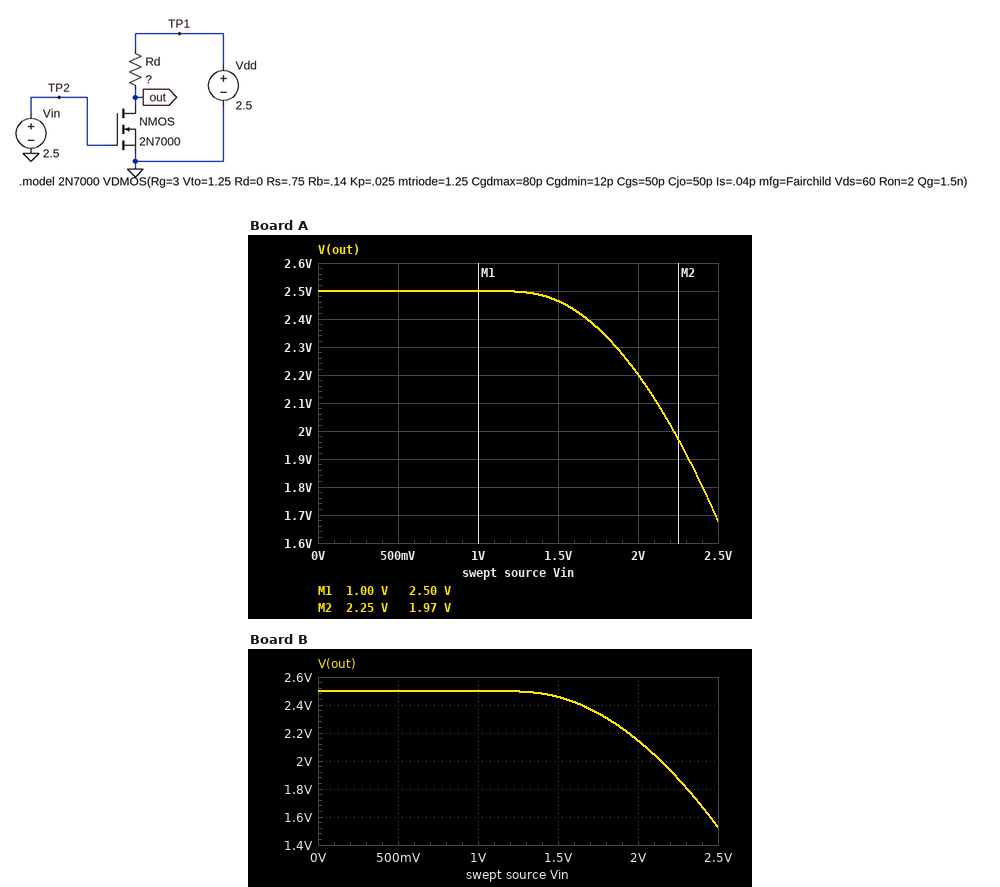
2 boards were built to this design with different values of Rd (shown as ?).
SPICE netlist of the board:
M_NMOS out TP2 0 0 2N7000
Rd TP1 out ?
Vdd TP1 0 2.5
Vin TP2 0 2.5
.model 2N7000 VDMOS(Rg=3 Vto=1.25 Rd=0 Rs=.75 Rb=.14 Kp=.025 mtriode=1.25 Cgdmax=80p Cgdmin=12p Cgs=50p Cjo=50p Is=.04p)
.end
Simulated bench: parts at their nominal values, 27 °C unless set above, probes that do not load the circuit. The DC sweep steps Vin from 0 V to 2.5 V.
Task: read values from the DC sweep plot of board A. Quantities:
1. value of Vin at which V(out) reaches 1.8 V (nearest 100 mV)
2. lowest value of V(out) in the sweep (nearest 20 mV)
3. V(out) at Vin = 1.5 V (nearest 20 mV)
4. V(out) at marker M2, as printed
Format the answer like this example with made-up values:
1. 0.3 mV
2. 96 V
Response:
1. 2.4 V
2. 1.68 V
3. 2.46 V
4. 1.97 V
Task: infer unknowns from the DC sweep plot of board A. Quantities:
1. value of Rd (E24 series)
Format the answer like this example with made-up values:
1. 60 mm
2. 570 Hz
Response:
1. 43 Ω
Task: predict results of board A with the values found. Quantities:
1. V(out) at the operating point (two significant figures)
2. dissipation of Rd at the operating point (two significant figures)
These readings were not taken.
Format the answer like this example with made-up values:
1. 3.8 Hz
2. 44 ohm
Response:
1. 1.7 V
2. 16 mW
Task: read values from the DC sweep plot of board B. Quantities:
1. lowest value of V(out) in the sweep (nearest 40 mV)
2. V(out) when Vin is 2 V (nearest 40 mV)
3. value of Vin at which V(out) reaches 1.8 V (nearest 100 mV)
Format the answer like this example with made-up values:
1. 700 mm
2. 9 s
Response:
1. 1.52 V
2. 2.16 V
3. 2.3 V
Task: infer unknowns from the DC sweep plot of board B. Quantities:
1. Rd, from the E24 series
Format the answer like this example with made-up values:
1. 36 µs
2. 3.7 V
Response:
1. 51 Ω
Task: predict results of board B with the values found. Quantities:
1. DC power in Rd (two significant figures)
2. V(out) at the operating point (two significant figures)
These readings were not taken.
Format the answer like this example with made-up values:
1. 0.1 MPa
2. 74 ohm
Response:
1. 19 mW
2. 1.5 V
